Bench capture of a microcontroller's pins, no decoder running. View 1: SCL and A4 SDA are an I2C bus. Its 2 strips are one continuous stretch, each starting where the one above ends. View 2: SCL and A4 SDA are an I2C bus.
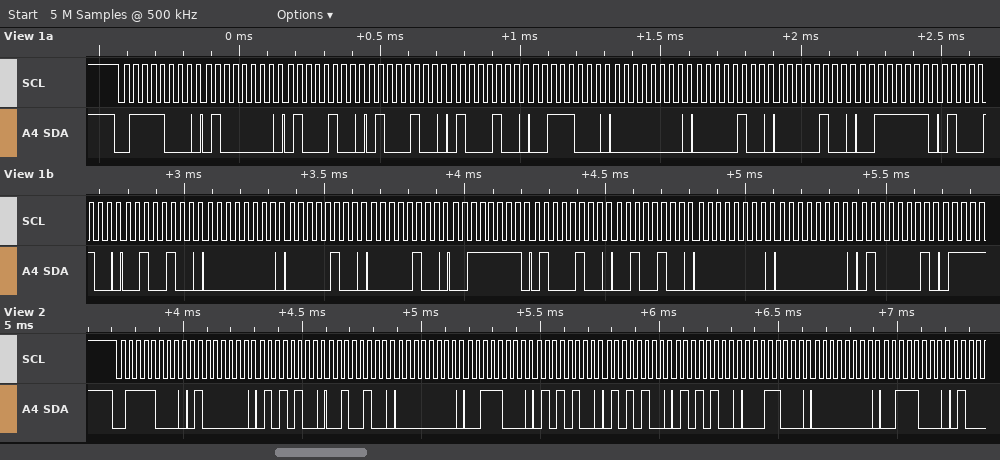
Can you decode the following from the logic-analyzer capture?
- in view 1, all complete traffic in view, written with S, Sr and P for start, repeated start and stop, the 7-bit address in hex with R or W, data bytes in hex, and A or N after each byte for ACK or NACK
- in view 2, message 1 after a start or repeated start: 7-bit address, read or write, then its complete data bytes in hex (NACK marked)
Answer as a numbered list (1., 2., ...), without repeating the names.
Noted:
1. S 3CW A 40 A 44 A 44 A 44 A 38 A 00 A 04 A 04 A 3F A 44 A 24 A 00 A 04 A 04 A 3F A 44 A 24 A 00 A 00 A 41 A
2. 0x3C write: 40 54 24 00 38 54 54 54 18 00 38
